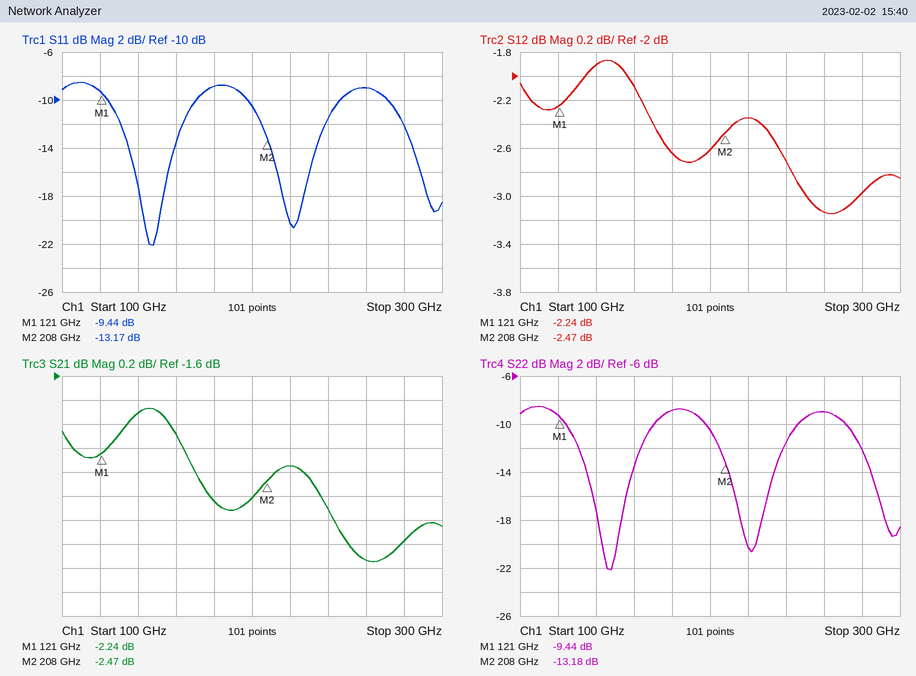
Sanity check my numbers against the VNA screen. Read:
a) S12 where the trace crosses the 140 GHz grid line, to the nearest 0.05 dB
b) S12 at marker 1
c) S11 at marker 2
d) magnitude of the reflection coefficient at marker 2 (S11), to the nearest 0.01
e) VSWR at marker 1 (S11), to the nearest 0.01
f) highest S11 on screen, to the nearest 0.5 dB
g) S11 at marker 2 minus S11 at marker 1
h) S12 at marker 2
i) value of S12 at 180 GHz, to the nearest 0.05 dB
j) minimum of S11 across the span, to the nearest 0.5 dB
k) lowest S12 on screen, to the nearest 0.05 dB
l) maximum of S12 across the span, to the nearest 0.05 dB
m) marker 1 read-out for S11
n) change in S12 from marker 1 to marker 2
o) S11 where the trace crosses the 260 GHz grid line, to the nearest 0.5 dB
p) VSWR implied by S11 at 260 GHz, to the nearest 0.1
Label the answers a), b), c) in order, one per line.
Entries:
a) -1.90 dB
b) -2.24 dB
c) -13.17 dB
d) 0.22
e) 2.02
f) -8.5 dB
g) -3.73 dB
h) -2.47 dB
i) -2.65 dB
j) -22.0 dB
k) -3.15 dB
l) -1.85 dB
m) -9.44 dB
n) -0.23 dB
o) -9.0 dB
p) 2.1
